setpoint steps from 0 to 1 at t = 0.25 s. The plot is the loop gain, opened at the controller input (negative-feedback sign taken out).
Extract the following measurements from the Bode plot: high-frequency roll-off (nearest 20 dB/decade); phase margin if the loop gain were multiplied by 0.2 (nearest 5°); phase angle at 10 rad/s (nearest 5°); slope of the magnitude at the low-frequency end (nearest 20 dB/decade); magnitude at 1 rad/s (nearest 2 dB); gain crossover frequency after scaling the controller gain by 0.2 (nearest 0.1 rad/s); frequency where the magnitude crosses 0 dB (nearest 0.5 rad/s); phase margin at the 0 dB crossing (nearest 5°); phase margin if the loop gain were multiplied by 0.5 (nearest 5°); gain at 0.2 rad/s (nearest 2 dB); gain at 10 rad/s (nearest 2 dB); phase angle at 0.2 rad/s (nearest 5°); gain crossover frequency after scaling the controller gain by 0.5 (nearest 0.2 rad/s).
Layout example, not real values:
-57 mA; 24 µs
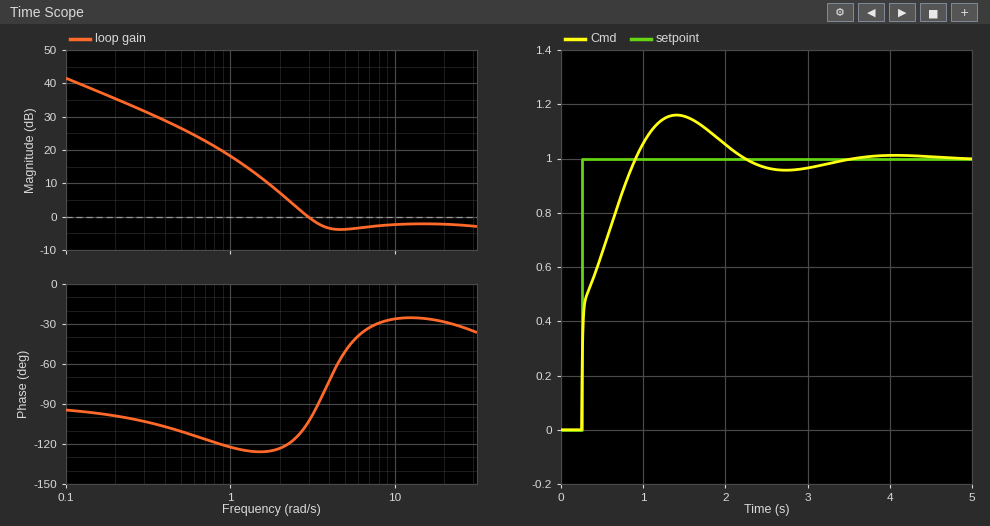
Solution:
0 dB/decade; 55°; -25°; -20 dB/decade; 18 dB; 1.3 rad/s; 3.0 rad/s; 75°; 60°; 36 dB; -2 dB; -100°; 2.2 rad/s
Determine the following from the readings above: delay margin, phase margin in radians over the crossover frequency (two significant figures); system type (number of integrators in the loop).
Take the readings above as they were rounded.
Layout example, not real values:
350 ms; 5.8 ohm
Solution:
0.44 s; 1
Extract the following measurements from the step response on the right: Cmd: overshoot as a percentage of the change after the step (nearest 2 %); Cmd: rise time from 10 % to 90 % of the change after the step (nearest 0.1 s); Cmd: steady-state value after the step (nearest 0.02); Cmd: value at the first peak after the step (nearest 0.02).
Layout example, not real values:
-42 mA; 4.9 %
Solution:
16 %; 0.5 s; 1.00; 1.16
